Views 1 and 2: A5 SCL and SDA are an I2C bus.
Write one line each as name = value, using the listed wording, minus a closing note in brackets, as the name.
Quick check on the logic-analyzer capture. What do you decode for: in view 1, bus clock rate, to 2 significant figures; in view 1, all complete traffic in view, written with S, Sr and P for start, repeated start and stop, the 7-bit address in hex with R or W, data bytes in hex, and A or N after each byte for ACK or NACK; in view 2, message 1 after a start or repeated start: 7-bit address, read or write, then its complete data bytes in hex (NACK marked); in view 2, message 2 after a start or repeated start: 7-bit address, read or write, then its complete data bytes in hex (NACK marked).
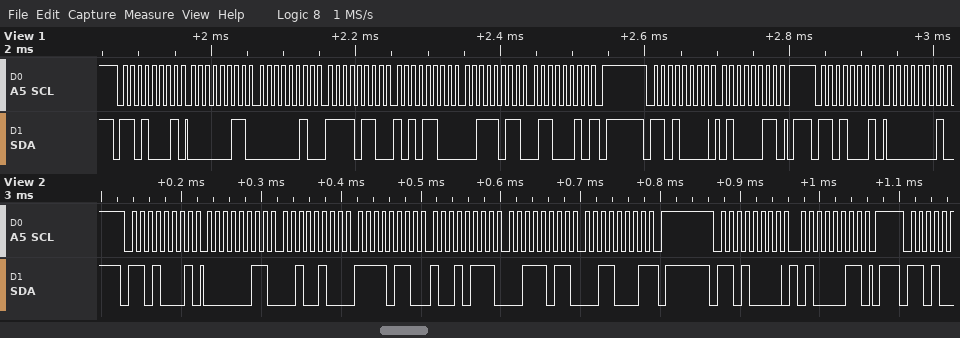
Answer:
in view 1, bus clock rate, to 2 significant figures = 100 kHz
in view 1, all complete traffic in view, written with S, Sr and P for start, repeated start and stop, the 7-bit address in hex with R or W, data bytes in hex, and A or N after each byte for ACK or NACK = S 68R A 03 A 02 A F6 A AC A 3B A 62 N P S 68W A 43 A P S 68R A 01 A
in view 2, message 1 after a start or repeated start: 7-bit address, read or write, then its complete data bytes in hex = 0x68 read: 03 24 F6 97 3B 31 NACK
in view 2, message 2 after a start or repeated start: 7-bit address, read or write, then its complete data bytes in hex = 0x68 write: 43
